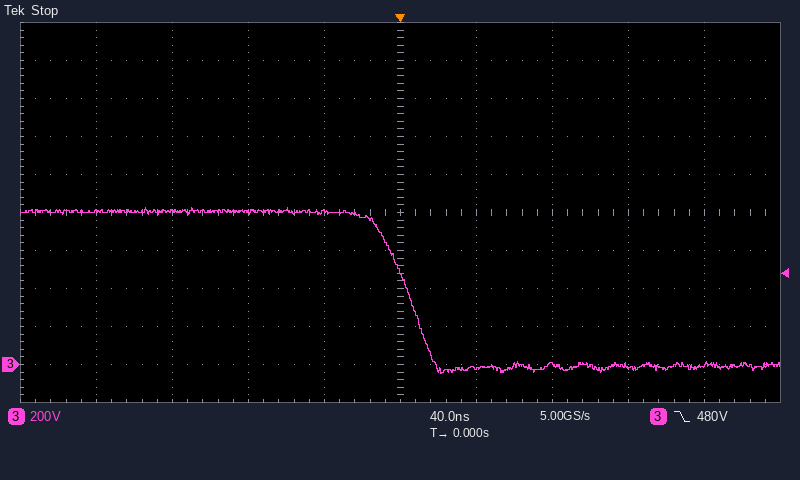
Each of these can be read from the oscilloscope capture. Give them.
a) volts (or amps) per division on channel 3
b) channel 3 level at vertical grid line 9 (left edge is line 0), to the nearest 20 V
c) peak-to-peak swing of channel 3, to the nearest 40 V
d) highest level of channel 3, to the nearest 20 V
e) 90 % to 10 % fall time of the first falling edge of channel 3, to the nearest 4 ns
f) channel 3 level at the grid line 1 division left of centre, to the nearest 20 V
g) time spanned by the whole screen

200 V
0 V
880 V
820 V
28 ns
800 V
400 ns
